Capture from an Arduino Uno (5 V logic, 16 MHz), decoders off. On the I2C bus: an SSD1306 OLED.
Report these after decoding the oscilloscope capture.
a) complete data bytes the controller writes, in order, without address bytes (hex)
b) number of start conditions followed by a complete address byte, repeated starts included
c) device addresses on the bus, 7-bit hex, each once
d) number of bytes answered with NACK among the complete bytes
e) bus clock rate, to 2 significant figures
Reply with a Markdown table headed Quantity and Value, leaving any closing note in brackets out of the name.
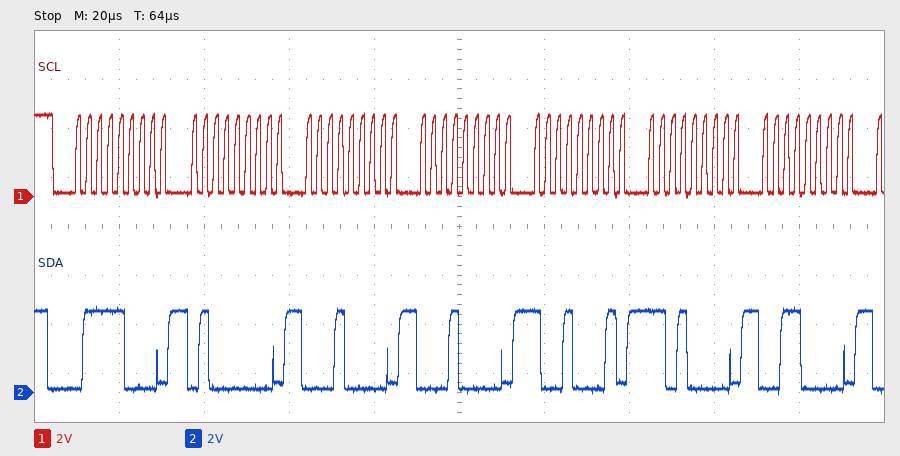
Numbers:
| Quantity | Value |
|---|---|
| complete data bytes the controller writes, in order, without address bytes | 40 10 10 91 D0 30 |
| number of start conditions followed by a complete address byte, repeated starts included | 1 |
| device addresses on the bus, 7-bit hex, each once | 0x3C |
| number of bytes answered with NACK among the complete bytes | 0 |
| bus clock rate, to 2 significant figures | 400 kHz |
